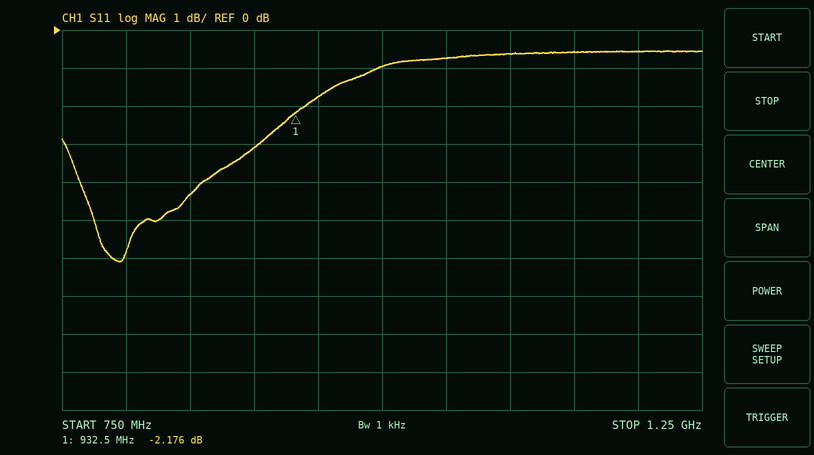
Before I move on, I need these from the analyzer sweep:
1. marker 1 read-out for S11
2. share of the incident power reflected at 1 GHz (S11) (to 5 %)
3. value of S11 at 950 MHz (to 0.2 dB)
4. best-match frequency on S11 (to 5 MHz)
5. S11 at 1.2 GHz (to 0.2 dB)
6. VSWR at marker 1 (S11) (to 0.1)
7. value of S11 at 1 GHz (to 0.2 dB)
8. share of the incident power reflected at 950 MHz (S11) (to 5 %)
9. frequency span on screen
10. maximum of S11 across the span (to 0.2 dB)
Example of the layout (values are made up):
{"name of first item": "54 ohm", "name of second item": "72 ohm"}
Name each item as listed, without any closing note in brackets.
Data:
{"marker 1 read-out for S11": "-2.176 dB", "share of the incident power reflected at 1 GHz (S11)": "80 %", "value of S11 at 950 MHz": "-1.8 dB", "best-match frequency on S11": "795 MHz", "S11 at 1.2 GHz": "-0.6 dB", "VSWR at marker 1 (S11)": "8.0", "value of S11 at 1 GHz": "-1.0 dB", "share of the incident power reflected at 950 MHz (S11)": "65 %", "frequency span on screen": "500 MHz", "maximum of S11 across the span": "-0.6 dB"}
